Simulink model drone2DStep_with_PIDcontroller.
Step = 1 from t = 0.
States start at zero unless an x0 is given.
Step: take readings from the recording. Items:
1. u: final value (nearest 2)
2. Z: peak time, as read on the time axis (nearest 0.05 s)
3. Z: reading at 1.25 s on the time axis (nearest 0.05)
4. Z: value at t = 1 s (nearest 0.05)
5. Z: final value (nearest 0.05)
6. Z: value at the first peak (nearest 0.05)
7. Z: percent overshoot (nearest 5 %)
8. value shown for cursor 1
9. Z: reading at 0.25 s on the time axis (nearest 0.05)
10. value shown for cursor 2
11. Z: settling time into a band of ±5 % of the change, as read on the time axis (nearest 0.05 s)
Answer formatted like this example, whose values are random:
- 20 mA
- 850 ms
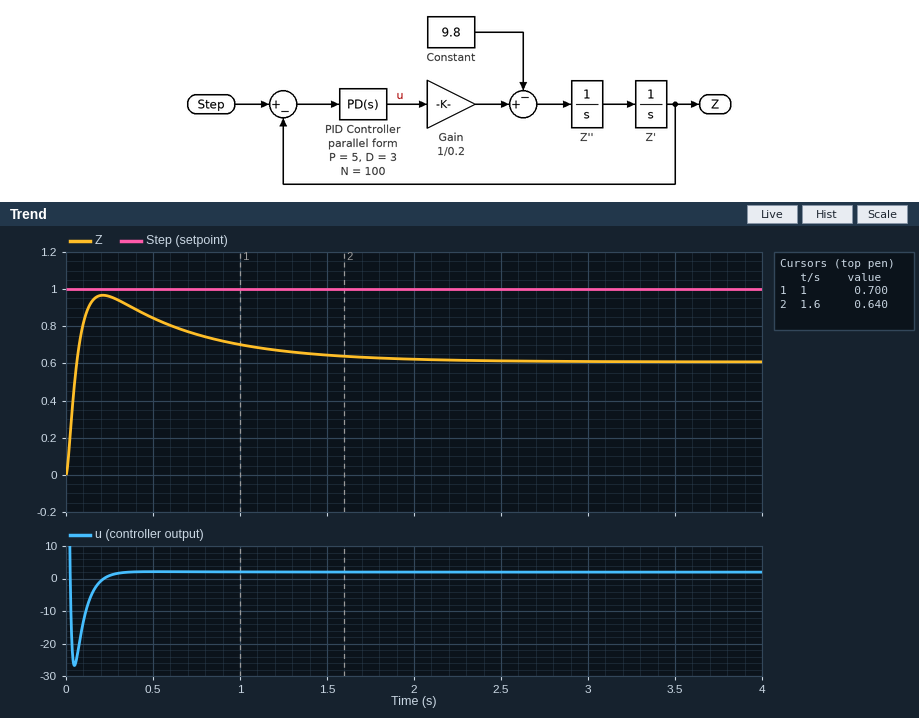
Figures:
- 2
- 0.20 s
- 0.65
- 0.70
- 0.60
- 0.95
- 60 %
- 0.700
- 0.95
- 0.640
- 1.60 s
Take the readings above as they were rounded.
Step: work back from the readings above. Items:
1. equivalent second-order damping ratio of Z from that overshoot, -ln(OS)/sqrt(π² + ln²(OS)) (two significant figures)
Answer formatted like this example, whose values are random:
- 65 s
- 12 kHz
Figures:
- 0.16
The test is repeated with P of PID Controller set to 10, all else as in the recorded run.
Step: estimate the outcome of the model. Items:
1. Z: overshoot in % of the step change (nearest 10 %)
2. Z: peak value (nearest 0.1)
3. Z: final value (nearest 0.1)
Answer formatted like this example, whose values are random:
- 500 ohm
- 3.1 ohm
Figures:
- 30 %
- 1.0
- 0.8
